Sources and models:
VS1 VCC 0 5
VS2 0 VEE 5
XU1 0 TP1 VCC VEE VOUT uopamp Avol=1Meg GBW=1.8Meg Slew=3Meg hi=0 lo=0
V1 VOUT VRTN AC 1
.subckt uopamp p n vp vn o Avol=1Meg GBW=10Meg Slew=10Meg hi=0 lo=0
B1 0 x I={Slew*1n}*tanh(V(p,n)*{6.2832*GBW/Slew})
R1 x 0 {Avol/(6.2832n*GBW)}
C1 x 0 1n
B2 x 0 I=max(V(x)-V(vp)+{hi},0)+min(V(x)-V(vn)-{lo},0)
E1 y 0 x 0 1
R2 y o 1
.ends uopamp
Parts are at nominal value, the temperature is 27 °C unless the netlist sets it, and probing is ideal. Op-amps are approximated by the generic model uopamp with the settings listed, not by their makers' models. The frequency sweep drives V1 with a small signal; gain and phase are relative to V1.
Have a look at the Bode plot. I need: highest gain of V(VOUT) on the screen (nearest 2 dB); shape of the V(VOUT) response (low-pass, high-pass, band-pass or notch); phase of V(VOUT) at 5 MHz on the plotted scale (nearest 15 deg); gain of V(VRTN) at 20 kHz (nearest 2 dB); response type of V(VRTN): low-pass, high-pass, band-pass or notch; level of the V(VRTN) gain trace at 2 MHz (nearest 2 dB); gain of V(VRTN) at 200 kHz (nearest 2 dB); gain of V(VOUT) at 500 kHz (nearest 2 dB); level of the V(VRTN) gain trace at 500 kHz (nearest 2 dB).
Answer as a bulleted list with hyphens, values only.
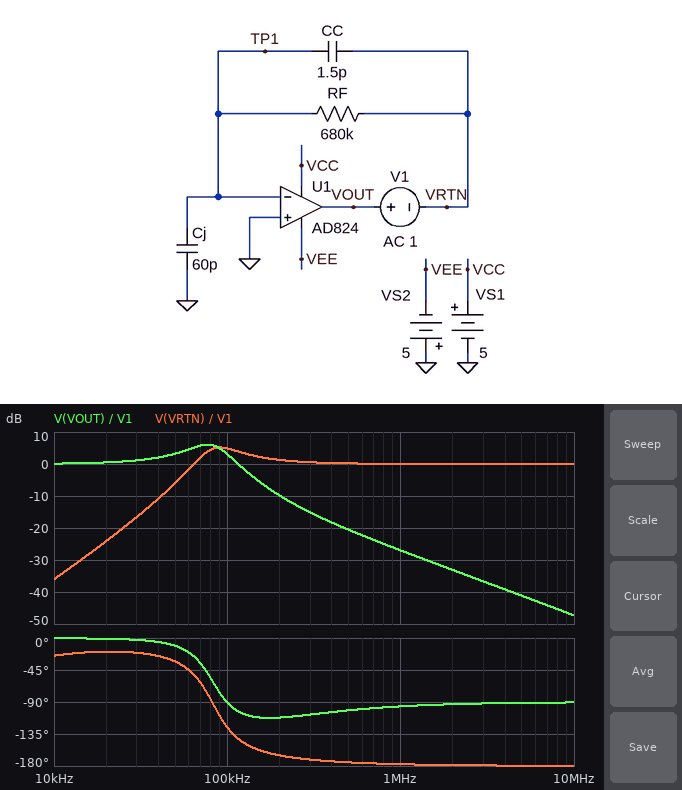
- 6 dB
- low-pass
- -90 deg
- -24 dB
- high-pass
- 0 dB
- 2 dB
- -20 dB
- 0 dB
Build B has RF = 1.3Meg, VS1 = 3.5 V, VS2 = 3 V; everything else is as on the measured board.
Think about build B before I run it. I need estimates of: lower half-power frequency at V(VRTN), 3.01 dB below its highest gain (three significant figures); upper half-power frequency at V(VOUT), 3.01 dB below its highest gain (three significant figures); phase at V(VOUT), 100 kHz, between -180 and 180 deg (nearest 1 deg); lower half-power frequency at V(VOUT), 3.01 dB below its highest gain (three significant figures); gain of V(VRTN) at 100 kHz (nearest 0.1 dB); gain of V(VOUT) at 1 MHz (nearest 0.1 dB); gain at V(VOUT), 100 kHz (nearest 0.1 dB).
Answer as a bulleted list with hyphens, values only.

- 50.3 kHz
- 76.2 kHz
- -94 deg
- 25.2 kHz
- 2.1 dB
- -27.1 dB
- -2.9 dB
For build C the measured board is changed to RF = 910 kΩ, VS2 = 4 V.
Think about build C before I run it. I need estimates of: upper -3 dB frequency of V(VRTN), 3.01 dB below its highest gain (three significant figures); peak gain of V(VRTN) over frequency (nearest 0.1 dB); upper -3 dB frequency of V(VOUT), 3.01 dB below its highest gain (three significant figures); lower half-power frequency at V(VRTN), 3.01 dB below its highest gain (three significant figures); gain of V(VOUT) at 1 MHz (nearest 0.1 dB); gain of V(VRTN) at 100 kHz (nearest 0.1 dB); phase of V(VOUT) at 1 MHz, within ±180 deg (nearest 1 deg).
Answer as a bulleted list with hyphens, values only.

- 174 kHz
- 4.2 dB
- 88.2 kHz
- 60.4 kHz
- -27.1 dB
- 3.4 dB
- -94 deg
